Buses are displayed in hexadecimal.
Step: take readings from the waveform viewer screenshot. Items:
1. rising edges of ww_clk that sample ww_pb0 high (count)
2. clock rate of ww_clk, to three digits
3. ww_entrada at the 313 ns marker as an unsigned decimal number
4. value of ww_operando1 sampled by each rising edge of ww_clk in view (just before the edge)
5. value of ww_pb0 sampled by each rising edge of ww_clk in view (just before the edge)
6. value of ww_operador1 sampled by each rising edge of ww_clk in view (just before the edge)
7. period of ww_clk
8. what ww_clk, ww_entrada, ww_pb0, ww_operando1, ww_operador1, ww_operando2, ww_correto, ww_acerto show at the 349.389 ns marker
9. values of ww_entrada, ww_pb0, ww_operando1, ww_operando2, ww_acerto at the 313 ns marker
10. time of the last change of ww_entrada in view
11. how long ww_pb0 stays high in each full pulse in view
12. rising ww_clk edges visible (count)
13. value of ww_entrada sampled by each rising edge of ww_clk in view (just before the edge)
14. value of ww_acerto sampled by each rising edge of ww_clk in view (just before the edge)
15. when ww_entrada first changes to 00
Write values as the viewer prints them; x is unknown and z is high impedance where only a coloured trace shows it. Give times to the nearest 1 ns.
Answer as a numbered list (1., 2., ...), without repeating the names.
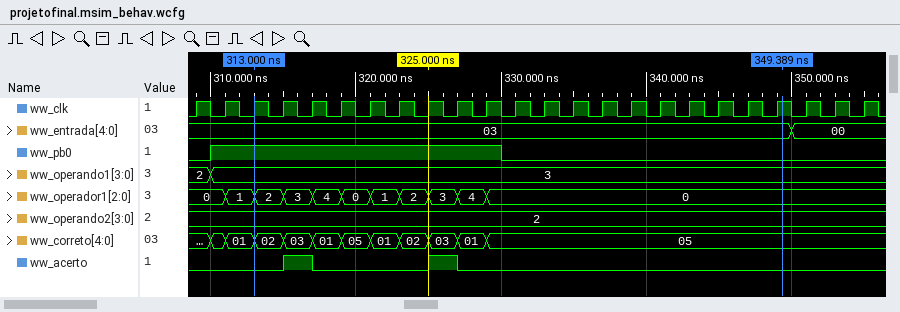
1. 10
2. 500 MHz
3. 3
4. 2, 3, 3, 3, 3, 3, 3, 3, 3, 3, 3, 3, 3, 3, 3, 3, 3, 3, 3, 3, 3, 3, 3, 3
5. 0 1 1 1 1 1 1 1 1 1 1 0 0 0 0 0 0 0 0 0 0 0 0 0
6. 0, 0, 1, 2, 3, 4, 0, 1, 2, 3, 4, 0, 0, 0, 0, 0, 0, 0, 0, 0, 0, 0, 0, 0
7. 2 ns
8. ww_clk=1, ww_entrada=03, ww_pb0=0, ww_operando1=3, ww_operador1=0, ww_operando2=2, ww_correto=05, ww_acerto=0
9. ww_entrada=03, ww_pb0=1, ww_operando1=3, ww_operando2=2, ww_acerto=0
10. 350 ns
11. 20 ns
12. 24
13. 03, 03, 03, 03, 03, 03, 03, 03, 03, 03, 03, 03, 03, 03, 03, 03, 03, 03, 03, 03, 03, 00, 00, 00
14. 0 0 0 0 1 0 0 0 0 1 0 0 0 0 0 0 0 0 0 0 0 0 0 0
15. 350 ns
